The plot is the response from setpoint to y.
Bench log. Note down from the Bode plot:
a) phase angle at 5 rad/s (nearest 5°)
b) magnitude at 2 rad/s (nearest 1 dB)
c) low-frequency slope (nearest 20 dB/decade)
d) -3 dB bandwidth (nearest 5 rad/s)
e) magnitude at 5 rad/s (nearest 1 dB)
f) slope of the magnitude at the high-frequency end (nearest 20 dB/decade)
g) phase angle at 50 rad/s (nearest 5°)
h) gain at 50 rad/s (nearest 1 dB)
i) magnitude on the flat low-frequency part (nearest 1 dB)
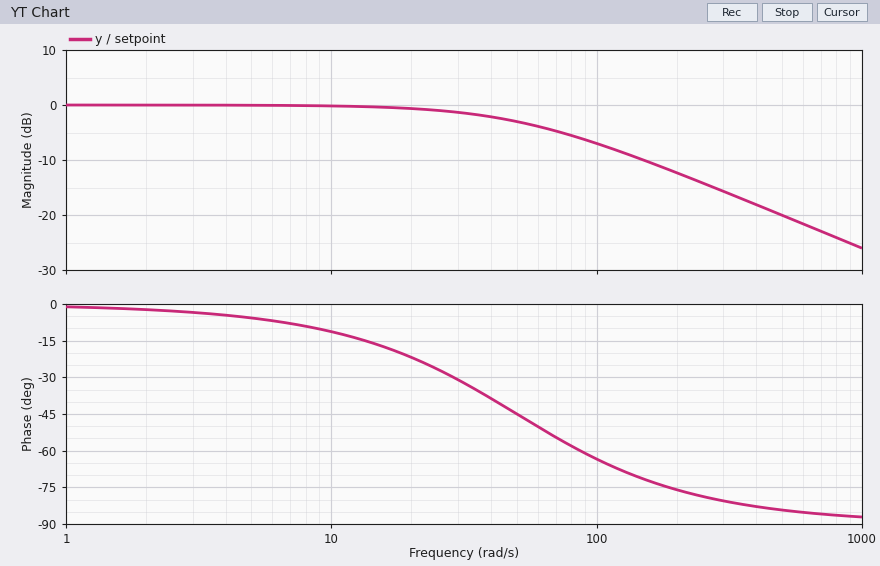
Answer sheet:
-5°
0 dB
0 dB/decade
50 rad/s
0 dB
-20 dB/decade
-45°
-3 dB
0 dB
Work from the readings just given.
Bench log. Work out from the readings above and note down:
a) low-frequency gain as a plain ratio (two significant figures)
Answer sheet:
1.0
